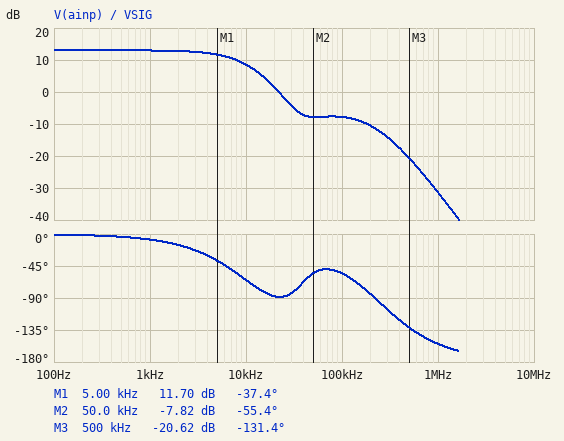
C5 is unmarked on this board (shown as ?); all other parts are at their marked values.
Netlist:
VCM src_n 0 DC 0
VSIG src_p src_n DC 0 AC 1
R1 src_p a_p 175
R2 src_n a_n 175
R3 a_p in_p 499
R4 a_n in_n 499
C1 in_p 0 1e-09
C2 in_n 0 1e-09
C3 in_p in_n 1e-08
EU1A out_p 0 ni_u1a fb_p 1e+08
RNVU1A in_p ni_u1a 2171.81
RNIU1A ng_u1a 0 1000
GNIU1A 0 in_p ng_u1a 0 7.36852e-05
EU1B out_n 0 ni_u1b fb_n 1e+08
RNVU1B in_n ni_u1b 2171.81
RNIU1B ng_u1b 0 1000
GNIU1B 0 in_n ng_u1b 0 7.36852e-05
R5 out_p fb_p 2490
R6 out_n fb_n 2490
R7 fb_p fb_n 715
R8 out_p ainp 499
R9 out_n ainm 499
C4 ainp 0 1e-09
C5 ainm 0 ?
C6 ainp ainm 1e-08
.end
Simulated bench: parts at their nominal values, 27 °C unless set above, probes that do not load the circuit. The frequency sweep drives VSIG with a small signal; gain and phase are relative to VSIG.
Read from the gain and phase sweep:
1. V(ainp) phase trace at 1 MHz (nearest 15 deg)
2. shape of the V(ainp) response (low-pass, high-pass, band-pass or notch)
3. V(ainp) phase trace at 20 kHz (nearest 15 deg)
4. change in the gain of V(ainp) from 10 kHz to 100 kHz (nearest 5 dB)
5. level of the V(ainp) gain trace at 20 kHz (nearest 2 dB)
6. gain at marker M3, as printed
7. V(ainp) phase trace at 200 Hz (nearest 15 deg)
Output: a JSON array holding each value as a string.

["-150 deg", "low-pass", "-90 deg", "-15 dB", "2 dB", "-20.62 dB", "0 deg"]
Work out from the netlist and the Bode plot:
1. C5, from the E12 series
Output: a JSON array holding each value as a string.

["1.8 nF"]
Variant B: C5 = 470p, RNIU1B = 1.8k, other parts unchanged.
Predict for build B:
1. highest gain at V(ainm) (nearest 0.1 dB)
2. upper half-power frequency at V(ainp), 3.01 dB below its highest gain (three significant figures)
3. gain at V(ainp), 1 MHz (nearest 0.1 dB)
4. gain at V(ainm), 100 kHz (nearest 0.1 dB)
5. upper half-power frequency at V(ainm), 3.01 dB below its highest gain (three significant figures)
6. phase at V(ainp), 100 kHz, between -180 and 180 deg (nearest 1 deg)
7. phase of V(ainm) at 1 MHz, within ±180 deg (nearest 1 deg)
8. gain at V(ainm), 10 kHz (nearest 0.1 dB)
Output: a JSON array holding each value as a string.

["10.8 dB", "7.95 kHz", "-26.8 dB", "-6.1 dB", "9.39 kHz", "-43 deg", "-143 deg", "7.5 dB"]
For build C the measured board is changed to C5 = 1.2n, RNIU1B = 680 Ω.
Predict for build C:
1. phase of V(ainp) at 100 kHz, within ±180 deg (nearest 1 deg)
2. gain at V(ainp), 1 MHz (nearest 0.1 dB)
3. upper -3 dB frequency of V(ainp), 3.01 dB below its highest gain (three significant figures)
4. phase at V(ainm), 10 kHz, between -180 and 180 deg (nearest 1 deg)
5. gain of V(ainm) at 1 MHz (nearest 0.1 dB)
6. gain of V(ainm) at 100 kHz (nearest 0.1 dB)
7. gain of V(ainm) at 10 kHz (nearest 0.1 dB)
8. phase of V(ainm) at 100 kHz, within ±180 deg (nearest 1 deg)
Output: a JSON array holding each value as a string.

["-50 deg", "-29.7 dB", "7.92 kHz", "93 deg", "-30.1 dB", "-6.5 dB", "7.5 dB", "-35 deg"]
